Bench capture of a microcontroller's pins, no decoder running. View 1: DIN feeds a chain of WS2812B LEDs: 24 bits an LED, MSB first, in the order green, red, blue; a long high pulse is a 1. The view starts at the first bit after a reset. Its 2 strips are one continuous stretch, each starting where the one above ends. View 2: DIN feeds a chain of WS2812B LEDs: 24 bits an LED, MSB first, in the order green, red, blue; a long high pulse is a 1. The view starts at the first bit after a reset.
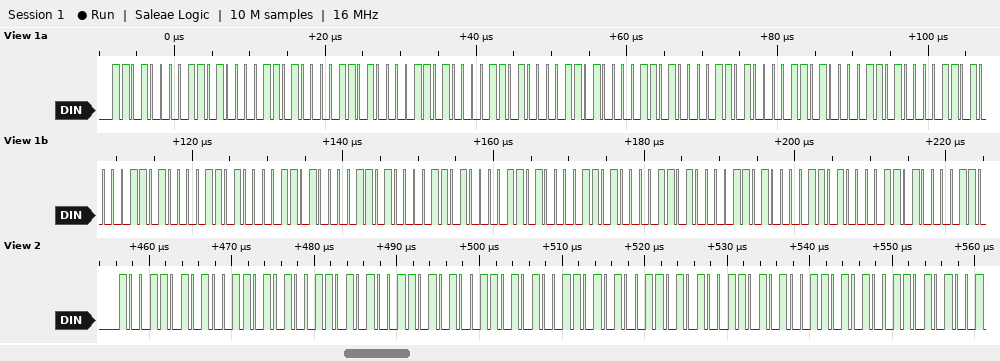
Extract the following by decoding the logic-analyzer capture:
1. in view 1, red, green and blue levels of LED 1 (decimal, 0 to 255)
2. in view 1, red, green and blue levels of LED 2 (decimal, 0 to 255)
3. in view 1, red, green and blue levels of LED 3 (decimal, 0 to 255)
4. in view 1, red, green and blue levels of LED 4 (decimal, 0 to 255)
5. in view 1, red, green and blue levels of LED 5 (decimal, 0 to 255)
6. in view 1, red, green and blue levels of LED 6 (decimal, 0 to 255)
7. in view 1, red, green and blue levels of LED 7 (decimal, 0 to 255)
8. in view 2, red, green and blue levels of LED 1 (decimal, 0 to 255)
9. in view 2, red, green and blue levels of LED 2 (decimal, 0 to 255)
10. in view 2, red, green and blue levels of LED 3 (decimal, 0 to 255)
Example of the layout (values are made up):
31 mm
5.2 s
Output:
208, 208, 208
208, 208, 208
208, 208, 208
208, 208, 208
208, 208, 208
208, 208, 208
208, 208, 208
154, 154, 154
154, 154, 154
154, 154, 154
